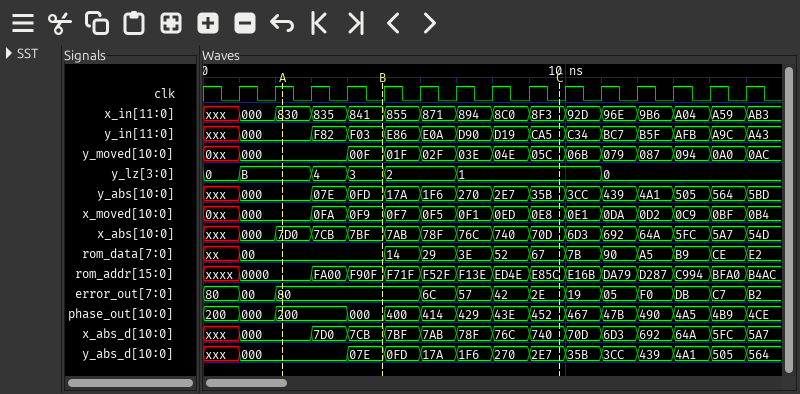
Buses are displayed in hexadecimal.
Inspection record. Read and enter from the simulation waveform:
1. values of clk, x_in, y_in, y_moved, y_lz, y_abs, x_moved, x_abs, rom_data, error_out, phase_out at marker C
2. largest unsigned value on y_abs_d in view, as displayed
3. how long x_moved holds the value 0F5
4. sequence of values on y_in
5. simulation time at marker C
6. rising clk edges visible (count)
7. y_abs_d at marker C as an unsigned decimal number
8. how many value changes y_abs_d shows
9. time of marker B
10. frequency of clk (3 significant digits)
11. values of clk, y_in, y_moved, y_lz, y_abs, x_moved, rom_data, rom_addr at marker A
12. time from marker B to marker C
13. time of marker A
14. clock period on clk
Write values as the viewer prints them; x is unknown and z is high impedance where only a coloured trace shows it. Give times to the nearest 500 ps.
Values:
clk=0, x_in=8F3, y_in=CA5, y_moved=05C, y_lz=1, y_abs=35B, x_moved=0E8, x_abs=70D, rom_data=67, error_out=2E, phase_out=452
564
1000 ps
xxx, 000, F82, F03, E86, E0A, D90, D19, CA5, C34, BC7, B5F, AFB, A9C, A43
10000 ps
15
743
13
5000 ps
1.00 GHz
clk=1, y_in=000, y_moved=000, y_lz=B, y_abs=000, x_moved=000, rom_data=00, rom_addr=0000
5000 ps
2000 ps
1000 ps
